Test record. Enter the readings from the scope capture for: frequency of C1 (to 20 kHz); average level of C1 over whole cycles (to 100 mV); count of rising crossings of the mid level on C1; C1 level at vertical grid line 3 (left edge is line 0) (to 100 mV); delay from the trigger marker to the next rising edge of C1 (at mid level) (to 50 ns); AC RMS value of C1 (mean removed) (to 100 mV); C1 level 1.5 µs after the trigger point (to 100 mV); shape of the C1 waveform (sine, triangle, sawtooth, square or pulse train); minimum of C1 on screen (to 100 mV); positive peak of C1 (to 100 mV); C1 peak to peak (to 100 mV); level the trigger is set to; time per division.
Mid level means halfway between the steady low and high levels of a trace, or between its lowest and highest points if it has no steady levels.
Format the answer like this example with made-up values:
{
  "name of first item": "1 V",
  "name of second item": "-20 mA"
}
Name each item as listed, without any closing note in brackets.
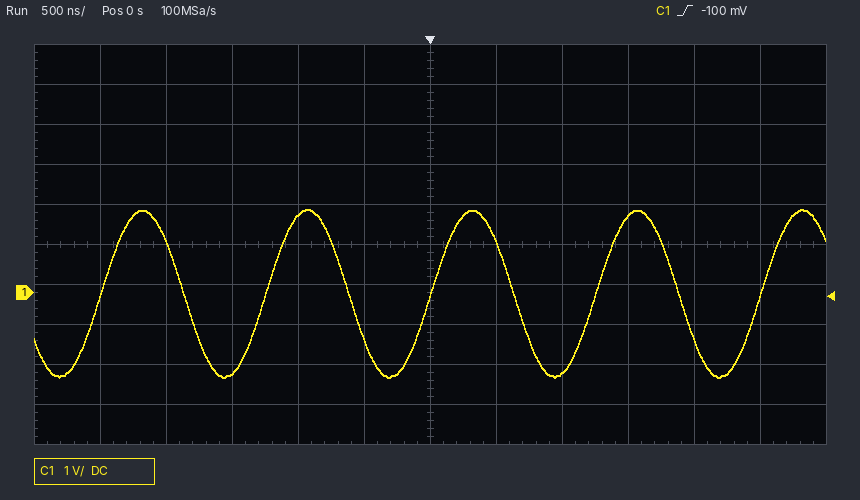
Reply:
{
  "frequency of C1": "800 kHz",
  "average level of C1 over whole cycles": "0.0 V",
  "count of rising crossings of the mid level on C1": "5",
  "C1 level at vertical grid line 3 (left edge is line 0)": "-2.0 V",
  "delay from the trigger marker to the next rising edge of C1 (at mid level)": "1.25 µs",
  "AC RMS value of C1 (mean removed)": "1.5 V",
  "C1 level 1.5 µs after the trigger point": "1.9 V",
  "shape of the C1 waveform": "sine",
  "minimum of C1 on screen": "-2.1 V",
  "positive peak of C1": "2.1 V",
  "C1 peak to peak": "4.2 V",
  "level the trigger is set to": "-100 mV",
  "time per division": "500 ns"
}
